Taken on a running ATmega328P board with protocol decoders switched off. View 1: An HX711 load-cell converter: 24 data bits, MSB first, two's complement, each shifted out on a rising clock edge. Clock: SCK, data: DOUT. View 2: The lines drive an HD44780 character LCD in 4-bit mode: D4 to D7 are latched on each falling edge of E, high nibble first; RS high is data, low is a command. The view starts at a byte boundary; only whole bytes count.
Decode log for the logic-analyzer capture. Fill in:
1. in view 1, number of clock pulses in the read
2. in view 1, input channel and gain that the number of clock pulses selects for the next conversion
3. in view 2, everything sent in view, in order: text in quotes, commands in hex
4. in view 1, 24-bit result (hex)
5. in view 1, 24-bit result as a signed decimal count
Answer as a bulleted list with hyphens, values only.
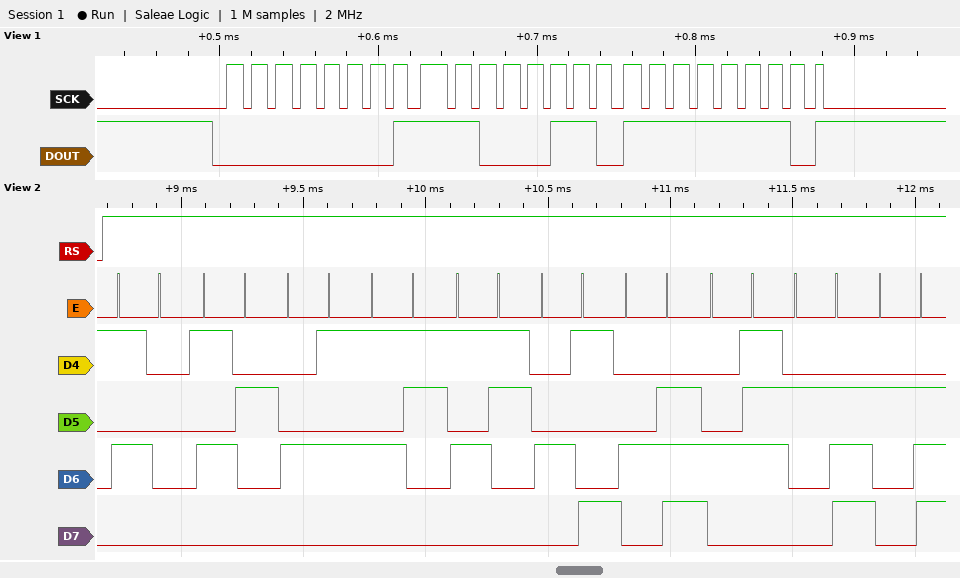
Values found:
- 25
- channel A, gain 128
- "PRESSING.."
- 0x01C6FE
- 116478
